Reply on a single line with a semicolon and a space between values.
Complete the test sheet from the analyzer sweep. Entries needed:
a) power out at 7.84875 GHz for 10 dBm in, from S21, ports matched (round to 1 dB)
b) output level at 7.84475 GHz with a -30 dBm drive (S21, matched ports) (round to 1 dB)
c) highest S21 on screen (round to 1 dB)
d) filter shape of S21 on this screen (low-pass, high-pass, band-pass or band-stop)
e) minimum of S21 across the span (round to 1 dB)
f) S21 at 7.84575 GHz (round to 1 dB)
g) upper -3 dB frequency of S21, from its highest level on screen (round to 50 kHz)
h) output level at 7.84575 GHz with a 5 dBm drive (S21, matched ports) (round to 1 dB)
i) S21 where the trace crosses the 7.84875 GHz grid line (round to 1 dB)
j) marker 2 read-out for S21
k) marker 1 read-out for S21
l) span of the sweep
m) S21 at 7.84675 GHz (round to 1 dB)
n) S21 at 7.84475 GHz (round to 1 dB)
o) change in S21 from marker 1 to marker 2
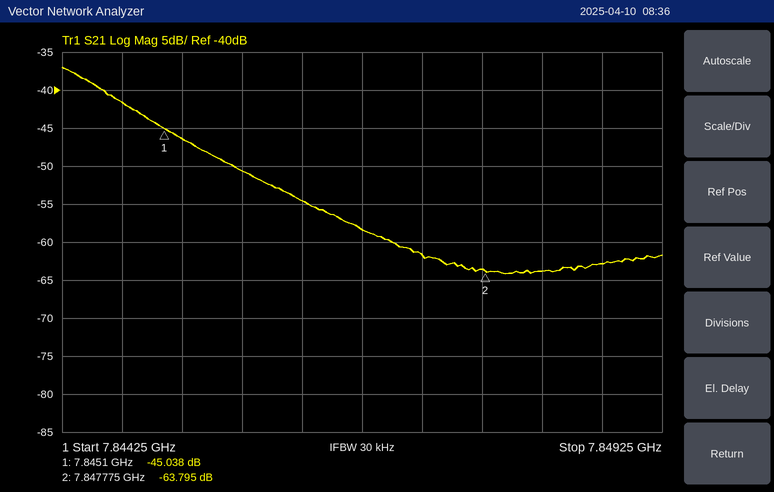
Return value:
-53 dBm; -72 dBm; -37 dB; low-pass; -64 dB; -51 dB; 7.84460 GHz; -46 dBm; -63 dB; -63.795 dB; -45.038 dB; 5 MHz; -58 dB; -42 dB; -18.757 dB
